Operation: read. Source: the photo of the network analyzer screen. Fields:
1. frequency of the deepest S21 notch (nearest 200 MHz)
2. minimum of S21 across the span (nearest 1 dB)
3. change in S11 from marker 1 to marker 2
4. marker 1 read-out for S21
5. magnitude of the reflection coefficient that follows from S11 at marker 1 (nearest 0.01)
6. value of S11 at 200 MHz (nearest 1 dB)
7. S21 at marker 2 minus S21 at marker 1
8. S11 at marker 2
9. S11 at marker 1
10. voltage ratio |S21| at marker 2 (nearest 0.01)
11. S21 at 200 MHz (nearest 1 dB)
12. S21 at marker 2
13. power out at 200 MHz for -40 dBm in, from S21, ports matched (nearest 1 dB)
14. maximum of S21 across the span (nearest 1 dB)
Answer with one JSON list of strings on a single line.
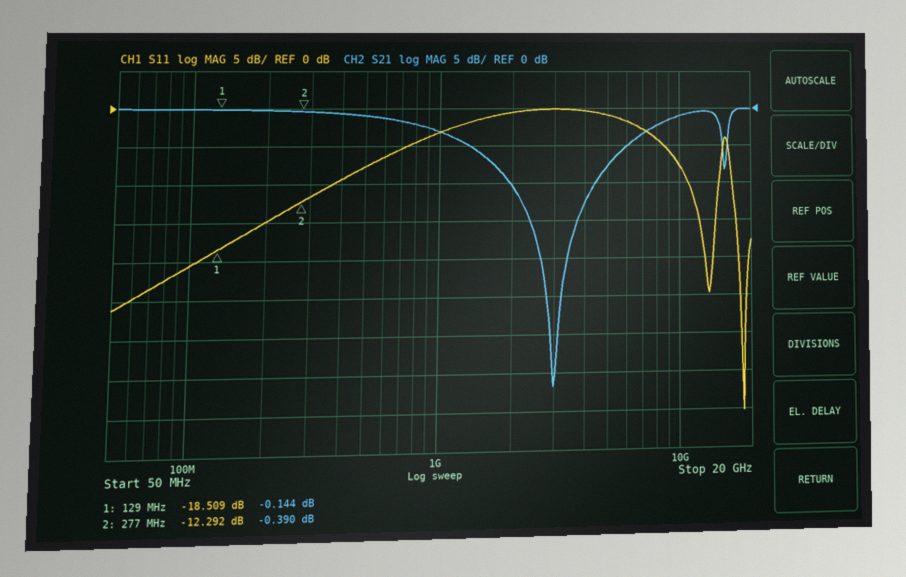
["3.0 GHz", "-37 dB", "6.217 dB", "-0.144 dB", "0.12", "-15 dB", "-0.246 dB", "-12.292 dB", "-18.509 dB", "0.96", "0 dB", "-0.390 dB", "-40 dBm", "0 dB"]
